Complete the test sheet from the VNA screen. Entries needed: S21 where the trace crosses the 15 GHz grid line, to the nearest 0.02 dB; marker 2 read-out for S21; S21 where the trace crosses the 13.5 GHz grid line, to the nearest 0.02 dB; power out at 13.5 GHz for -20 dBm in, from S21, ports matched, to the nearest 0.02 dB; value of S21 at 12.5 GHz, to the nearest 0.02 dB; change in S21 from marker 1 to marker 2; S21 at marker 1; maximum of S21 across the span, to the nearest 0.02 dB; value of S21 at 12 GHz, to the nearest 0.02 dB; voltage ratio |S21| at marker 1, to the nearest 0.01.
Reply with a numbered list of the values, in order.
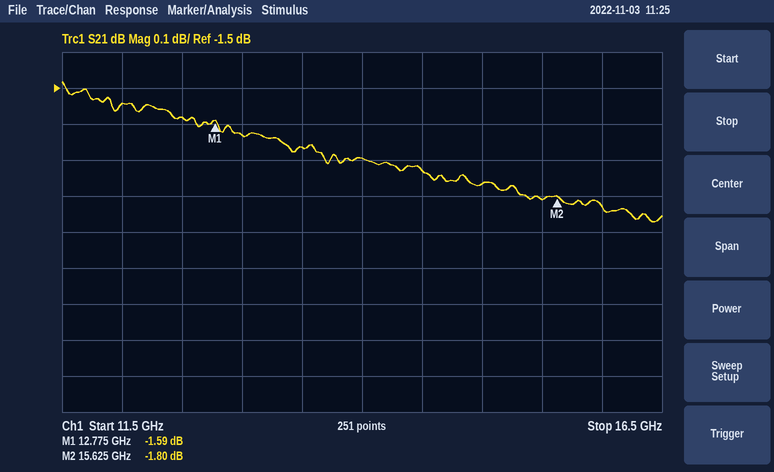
1. -1.76 dB
2. -1.80 dB
3. -1.66 dB
4. -21.66 dBm
5. -1.58 dB
6. -0.21 dB
7. -1.59 dB
8. -1.48 dB
9. -1.54 dB
10. 0.83
